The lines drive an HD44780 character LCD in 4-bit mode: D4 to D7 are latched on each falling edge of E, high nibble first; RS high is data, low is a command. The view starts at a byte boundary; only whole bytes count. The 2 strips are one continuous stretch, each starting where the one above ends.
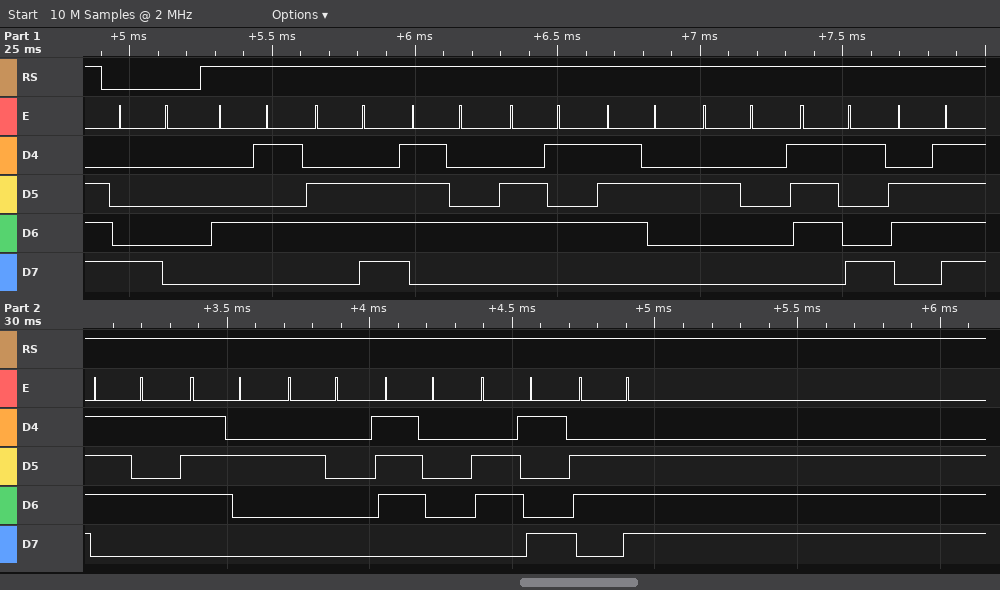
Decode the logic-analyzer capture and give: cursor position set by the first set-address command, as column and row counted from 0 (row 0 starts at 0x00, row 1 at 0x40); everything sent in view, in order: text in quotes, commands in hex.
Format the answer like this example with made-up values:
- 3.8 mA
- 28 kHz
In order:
- column 0, row 0
- 0x80 "Enter your pin"
